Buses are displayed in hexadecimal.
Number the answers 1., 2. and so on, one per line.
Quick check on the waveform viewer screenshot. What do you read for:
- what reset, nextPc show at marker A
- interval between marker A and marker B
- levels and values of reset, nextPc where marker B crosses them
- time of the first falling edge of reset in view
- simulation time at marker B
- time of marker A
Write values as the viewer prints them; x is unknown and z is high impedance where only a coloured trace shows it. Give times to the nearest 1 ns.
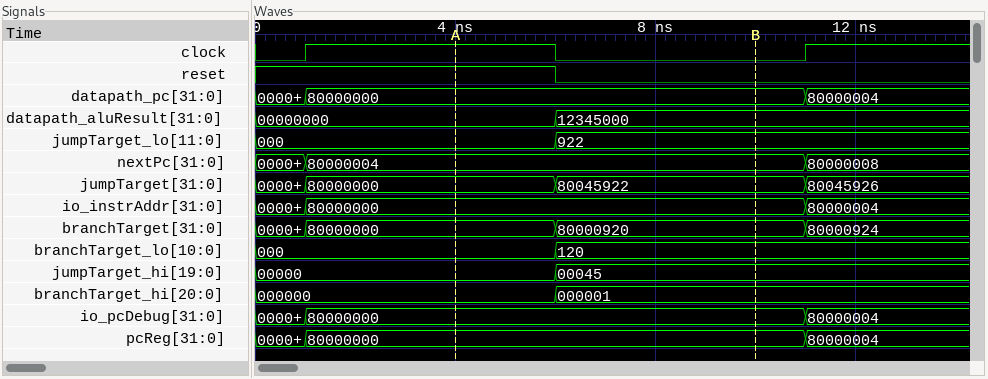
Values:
1. reset=1, nextPc=80000004
2. 6 ns
3. reset=0, nextPc=80000004
4. 6 ns
5. 10 ns
6. 4 ns
